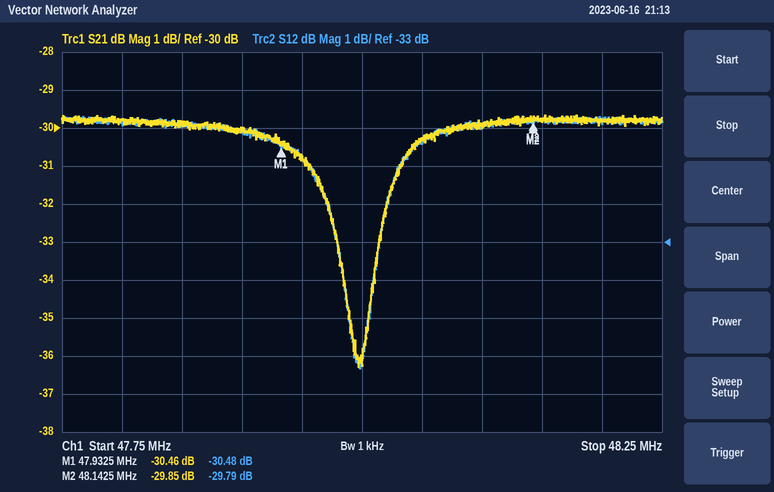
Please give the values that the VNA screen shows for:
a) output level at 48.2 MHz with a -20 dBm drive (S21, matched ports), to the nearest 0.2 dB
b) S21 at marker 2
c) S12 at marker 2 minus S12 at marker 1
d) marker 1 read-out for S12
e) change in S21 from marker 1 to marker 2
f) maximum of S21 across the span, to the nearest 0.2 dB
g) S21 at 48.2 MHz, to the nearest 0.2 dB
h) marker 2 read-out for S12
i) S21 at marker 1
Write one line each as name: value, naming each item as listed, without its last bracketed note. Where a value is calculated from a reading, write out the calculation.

output level at 48.2 MHz with a -20 dBm drive (S21, matched ports), to the nearest 0.2 dB: -20 dBm + (-29.8 dB) = -49.8 dBm
S21 at marker 2: -29.85 dB
S12 at marker 2 minus S12 at marker 1: -29.79 − (-30.48) = 0.69 dB
marker 1 read-out for S12: -30.48 dB
change in S21 from marker 1 to marker 2: -29.85 − (-30.46) = 0.61 dB
maximum of S21 across the span, to the nearest 0.2 dB: -29.6 dB
S21 at 48.2 MHz, to the nearest 0.2 dB: -29.8 dB
marker 2 read-out for S12: -29.79 dB
S21 at marker 1: -30.46 dB
